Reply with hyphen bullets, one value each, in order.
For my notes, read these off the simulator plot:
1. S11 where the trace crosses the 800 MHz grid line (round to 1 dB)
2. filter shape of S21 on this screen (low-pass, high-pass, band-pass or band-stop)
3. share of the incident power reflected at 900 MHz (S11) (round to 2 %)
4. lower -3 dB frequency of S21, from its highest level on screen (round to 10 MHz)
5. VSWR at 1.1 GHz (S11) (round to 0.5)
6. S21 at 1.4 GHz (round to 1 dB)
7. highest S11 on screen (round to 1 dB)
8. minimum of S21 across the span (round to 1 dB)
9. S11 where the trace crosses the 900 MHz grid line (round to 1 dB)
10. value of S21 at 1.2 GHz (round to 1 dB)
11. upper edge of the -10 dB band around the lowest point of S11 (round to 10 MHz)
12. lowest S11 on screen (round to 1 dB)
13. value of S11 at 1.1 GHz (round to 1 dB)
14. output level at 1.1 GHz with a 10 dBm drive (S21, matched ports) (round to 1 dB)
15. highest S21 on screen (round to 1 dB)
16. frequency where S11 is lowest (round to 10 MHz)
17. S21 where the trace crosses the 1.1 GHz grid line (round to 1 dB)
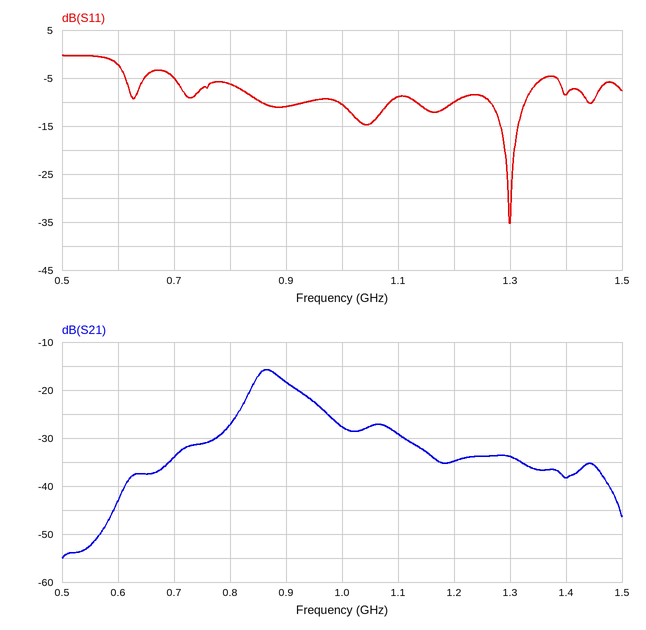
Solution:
- -6 dB
- band-pass
- 8 %
- 840 MHz
- 2.0
- -38 dB
- 0 dB
- -55 dB
- -11 dB
- -35 dB
- 1.33 GHz
- -35 dB
- -9 dB
- -19 dBm
- -16 dB
- 1.30 GHz
- -29 dB
